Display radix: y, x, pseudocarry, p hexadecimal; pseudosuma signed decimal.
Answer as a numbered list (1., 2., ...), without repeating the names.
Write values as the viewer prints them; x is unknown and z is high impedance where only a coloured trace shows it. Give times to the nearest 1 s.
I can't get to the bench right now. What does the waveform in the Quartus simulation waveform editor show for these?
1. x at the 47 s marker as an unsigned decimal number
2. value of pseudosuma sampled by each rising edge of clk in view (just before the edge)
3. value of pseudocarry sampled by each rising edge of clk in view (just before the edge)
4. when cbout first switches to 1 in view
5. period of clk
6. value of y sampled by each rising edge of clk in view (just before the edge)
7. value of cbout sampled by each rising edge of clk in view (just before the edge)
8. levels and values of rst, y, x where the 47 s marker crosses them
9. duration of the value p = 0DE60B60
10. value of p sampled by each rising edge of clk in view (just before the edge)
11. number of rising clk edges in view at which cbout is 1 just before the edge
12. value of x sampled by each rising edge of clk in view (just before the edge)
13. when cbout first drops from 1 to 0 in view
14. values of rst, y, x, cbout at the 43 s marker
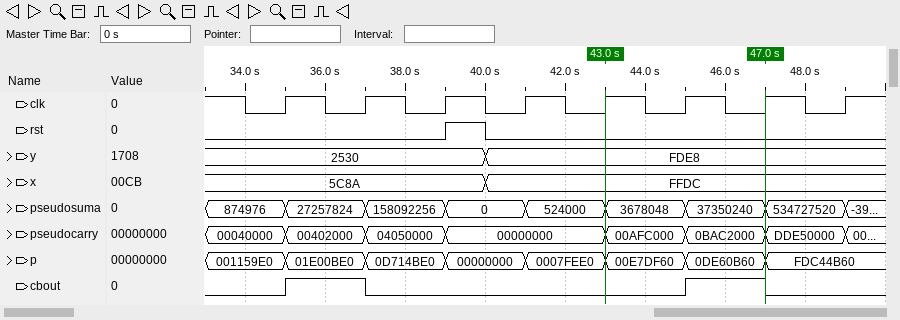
1. 65500
2. 874976, 27257824, 158092256, 0, 524000, 3678048, 37350240, 534727520
3. 00040000, 00402000, 04050000, 00000000, 00000000, 00AFC000, 0BAC2000, DDE50000
4. 35 s
5. 2 s
6. 2530, 2530, 2530, FDE8, FDE8, FDE8, FDE8, FDE8
7. 0 1 0 0 0 0 1 0
8. rst=0, y=FDE8, x=FFDC
9. 2 s
10. 001159E0, 01E00BE0, 0D714BE0, 00000000, 0007FEE0, 00E7DF60, 0DE60B60, FDC44B60
11. 2
12. 5C8A, 5C8A, 5C8A, FFDC, FFDC, FFDC, FFDC, FFDC
13. 37 s
14. rst=0, y=FDE8, x=FFDC, cbout=0
